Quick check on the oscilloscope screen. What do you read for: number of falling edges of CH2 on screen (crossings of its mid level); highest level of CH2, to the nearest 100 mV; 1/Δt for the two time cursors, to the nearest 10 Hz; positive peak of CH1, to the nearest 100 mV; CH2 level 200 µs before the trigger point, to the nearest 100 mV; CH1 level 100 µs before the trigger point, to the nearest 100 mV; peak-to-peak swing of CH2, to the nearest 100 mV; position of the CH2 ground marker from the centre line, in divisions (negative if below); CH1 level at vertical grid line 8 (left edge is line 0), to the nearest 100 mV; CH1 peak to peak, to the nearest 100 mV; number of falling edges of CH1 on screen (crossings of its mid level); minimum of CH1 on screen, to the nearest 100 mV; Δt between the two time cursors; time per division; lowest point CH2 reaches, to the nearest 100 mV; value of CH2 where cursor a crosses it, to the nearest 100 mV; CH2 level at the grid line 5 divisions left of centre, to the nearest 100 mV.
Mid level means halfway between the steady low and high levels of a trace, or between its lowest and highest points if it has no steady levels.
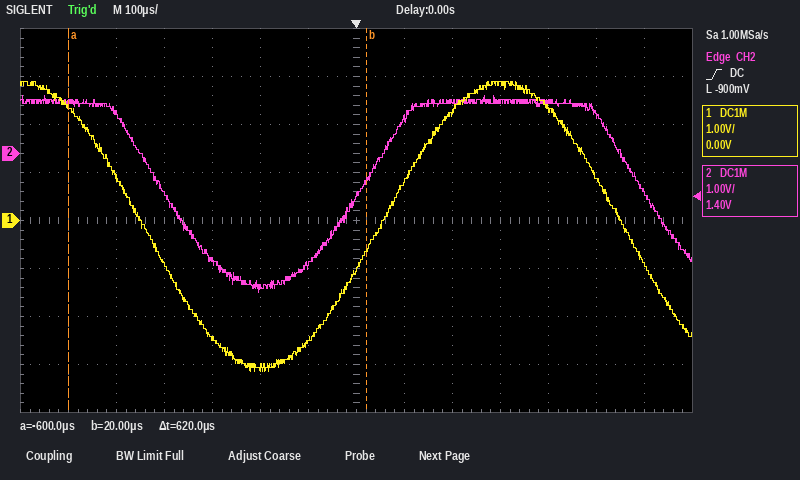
2
1.2 V
1.61 kHz
2.9 V
-2.8 V
-2.5 V
4.1 V
+1.4 div
800 mV
6.0 V
2
-3.1 V
620 µs
100 µs
-2.9 V
1.1 V
800 mV
